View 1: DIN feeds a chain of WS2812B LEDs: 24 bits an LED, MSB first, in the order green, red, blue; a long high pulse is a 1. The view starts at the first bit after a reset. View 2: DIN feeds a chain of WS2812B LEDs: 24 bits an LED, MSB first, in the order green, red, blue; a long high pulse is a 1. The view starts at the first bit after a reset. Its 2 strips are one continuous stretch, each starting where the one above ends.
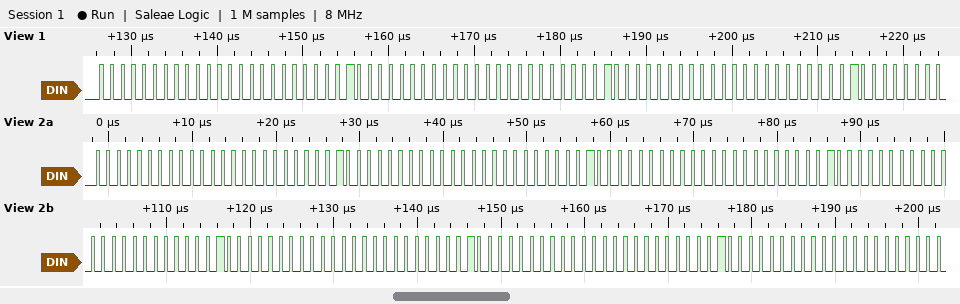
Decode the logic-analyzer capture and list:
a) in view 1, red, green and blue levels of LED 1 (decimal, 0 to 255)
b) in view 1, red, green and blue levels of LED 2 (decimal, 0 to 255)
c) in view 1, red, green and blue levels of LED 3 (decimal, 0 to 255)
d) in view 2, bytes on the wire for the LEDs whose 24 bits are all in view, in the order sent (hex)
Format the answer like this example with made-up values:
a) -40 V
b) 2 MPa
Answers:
a) 0, 0, 1
b) 0, 0, 1
c) 0, 0, 2
d) 00 00 01 00 00 01 00 00 02 00 00 02 00 00 02 00 00 02
